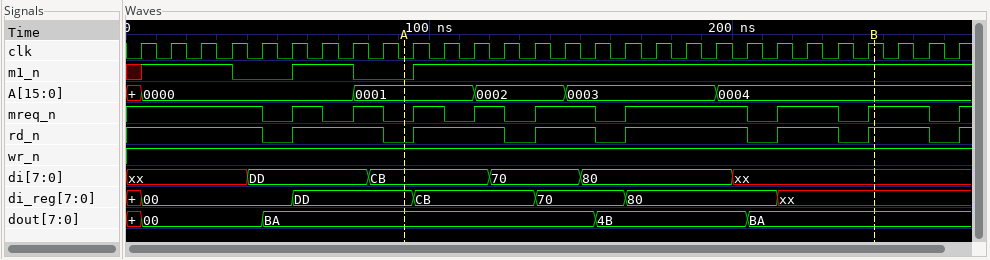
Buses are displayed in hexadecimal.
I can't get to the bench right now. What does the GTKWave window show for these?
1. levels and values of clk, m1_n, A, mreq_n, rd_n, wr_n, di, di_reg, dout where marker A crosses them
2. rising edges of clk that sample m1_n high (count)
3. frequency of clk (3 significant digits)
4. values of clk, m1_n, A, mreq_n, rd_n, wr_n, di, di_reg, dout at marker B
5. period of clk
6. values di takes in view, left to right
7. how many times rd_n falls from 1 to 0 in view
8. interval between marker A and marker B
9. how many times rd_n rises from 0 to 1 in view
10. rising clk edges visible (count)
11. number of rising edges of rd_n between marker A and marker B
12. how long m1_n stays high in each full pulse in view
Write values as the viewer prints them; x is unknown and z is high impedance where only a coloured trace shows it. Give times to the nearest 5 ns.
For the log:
clk=0, m1_n=0, A=0001, mreq_n=0, rd_n=0, wr_n=1, di=CB, di_reg=DD, dout=BA
23
100 MHz
clk=1, m1_n=1, A=0004, mreq_n=1, rd_n=1, wr_n=1, di=xx, di_reg=xx, dout=BA
10 ns
xx, DD, CB, 70, 80, xx
7
155 ns
7
28
5
20 ns
